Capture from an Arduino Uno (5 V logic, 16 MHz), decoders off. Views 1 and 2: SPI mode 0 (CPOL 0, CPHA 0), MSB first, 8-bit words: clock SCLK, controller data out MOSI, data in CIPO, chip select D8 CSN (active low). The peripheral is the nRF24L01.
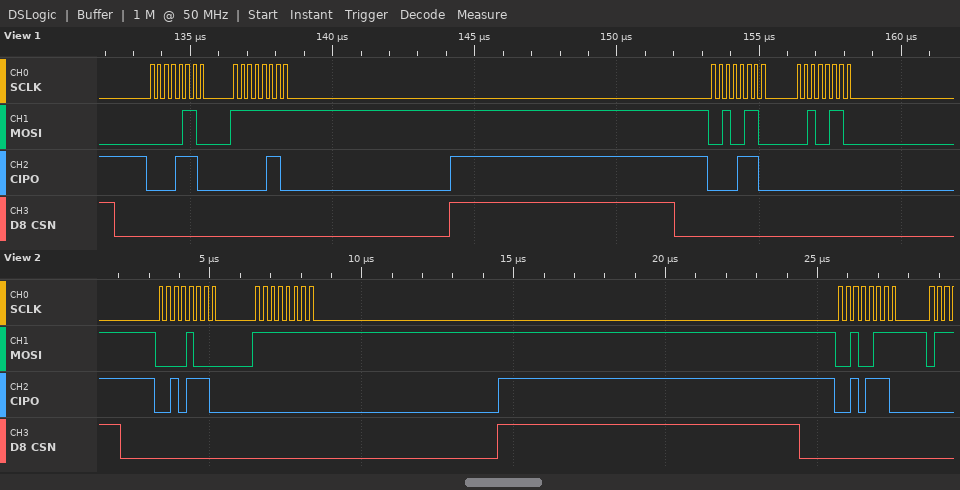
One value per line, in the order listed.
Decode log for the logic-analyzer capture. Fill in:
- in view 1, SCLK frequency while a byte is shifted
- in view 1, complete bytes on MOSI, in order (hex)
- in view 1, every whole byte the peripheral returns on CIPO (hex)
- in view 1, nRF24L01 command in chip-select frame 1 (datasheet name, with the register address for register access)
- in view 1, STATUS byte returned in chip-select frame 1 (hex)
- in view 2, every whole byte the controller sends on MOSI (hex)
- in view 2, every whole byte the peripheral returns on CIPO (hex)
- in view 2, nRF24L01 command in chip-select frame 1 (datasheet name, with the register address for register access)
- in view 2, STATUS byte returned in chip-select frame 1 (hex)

4 MHz
06 FF 26 26
0E 06 0E 00
R_REGISTER 0x06
0x0E
08 FF 27
2E 00 2E
R_REGISTER 0x08
0x2E
